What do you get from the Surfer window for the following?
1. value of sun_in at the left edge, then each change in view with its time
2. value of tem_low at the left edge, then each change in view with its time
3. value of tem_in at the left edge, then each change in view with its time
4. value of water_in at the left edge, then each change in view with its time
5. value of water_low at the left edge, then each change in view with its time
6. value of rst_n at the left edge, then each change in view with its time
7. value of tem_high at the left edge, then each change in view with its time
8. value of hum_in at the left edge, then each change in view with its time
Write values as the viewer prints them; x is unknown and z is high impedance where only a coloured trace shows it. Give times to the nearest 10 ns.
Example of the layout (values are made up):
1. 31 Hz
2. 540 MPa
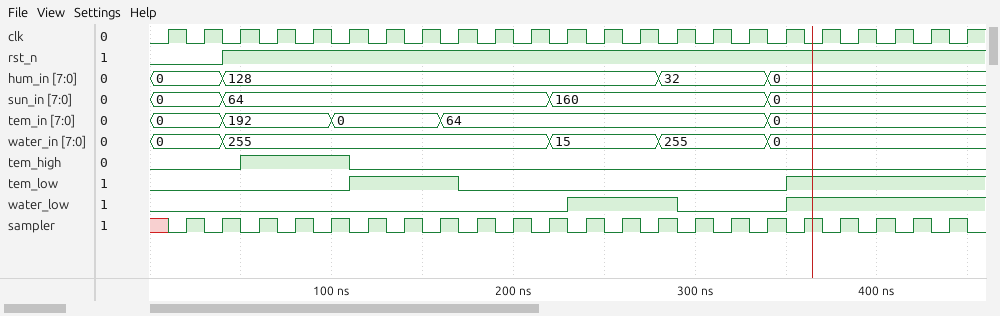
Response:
1. 0, 64 at 40 ns, 160 at 220 ns, 0 at 340 ns
2. 0, 1 at 110 ns, 0 at 170 ns, 1 at 350 ns
3. 0, 192 at 40 ns, 0 at 100 ns, 64 at 160 ns, 0 at 340 ns
4. 0, 255 at 40 ns, 15 at 220 ns, 255 at 280 ns, 0 at 340 ns
5. 0, 1 at 230 ns, 0 at 290 ns, 1 at 350 ns
6. 0, 1 at 40 ns
7. 0, 1 at 50 ns, 0 at 110 ns
8. 0, 128 at 40 ns, 32 at 280 ns, 0 at 340 ns
